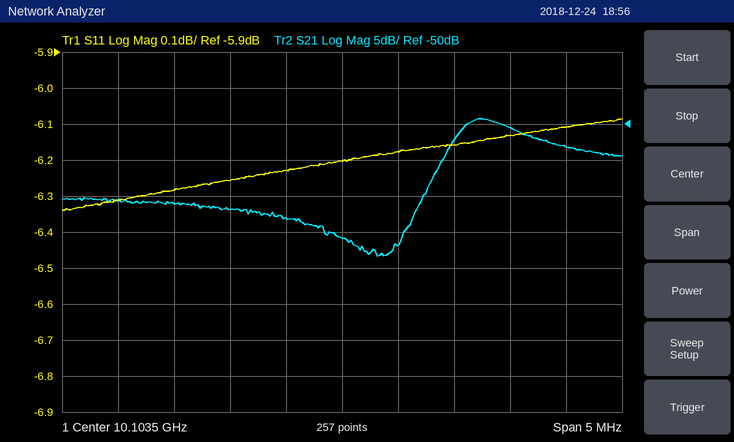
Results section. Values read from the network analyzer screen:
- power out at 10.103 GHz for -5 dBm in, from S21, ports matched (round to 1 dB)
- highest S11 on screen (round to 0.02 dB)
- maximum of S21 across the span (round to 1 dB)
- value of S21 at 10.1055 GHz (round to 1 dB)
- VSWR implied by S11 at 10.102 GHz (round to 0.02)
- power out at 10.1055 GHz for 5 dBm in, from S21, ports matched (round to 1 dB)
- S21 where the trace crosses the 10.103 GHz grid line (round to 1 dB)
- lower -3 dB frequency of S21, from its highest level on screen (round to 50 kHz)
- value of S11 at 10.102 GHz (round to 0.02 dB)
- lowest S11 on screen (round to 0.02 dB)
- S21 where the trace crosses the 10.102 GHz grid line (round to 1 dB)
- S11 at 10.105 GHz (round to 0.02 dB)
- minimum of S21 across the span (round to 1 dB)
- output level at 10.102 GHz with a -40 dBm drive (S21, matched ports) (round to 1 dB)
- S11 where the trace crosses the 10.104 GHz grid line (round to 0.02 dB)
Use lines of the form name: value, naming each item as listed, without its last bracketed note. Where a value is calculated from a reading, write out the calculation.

power out at 10.103 GHz for -5 dBm in, from S21, ports matched: -5 dBm + (-63 dB) = -68 dBm
highest S11 on screen: -6.08 dB
maximum of S21 across the span: -49 dB
value of S21 at 10.1055 GHz: -53 dB
VSWR implied by S11 at 10.102 GHz: |Γ| = 10^(-6.28/20) = 0.4853; VSWR = (1 + 0.4853)/(1 − 0.4853) ≈ 2.89, so 2.88 to the nearest 0.02
power out at 10.1055 GHz for 5 dBm in, from S21, ports matched: 5 dBm + (-53 dB) = -48 dBm
S21 where the trace crosses the 10.103 GHz grid line: -63 dB
lower -3 dB frequency of S21, from its highest level on screen: 10.10450 GHz
value of S11 at 10.102 GHz: -6.28 dB
lowest S11 on screen: -6.34 dB
S21 where the trace crosses the 10.102 GHz grid line: -61 dB
S11 at 10.105 GHz: -6.14 dB
minimum of S21 across the span: -68 dB
output level at 10.102 GHz with a -40 dBm drive (S21, matched ports): -40 dBm + (-61 dB) = -101 dBm
S11 where the trace crosses the 10.104 GHz grid line: -6.18 dB
